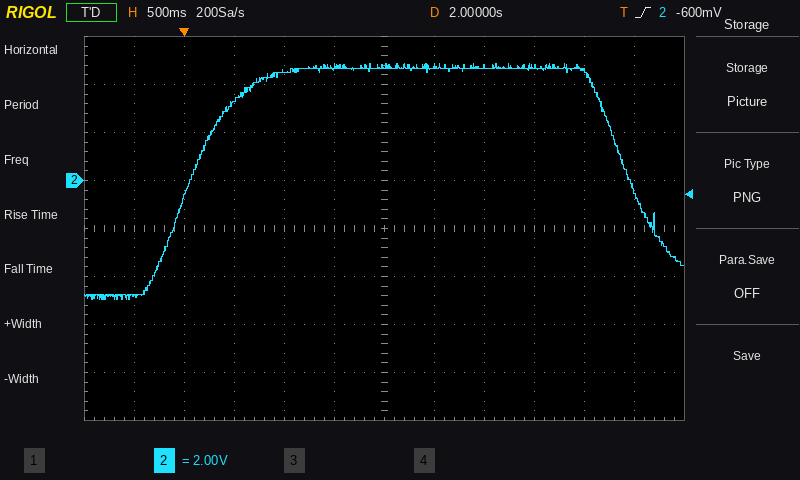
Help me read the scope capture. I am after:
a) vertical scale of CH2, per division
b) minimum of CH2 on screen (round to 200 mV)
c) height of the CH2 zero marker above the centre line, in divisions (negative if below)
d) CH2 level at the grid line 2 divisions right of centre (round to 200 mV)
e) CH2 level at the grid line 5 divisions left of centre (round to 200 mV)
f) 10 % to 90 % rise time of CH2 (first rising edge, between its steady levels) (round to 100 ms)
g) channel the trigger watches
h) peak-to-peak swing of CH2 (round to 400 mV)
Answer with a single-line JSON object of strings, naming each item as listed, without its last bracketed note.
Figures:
{"vertical scale of CH2, per division": "2 V", "minimum of CH2 on screen": "-5.0 V", "height of the CH2 zero marker above the centre line, in divisions": "+1.0 div", "CH2 level at the grid line 2 divisions right of centre": "4.8 V", "CH2 level at the grid line 5 divisions left of centre": "-4.8 V", "10 % to 90 % rise time of CH2 (first rising edge, between its steady levels)": "900 ms", "channel the trigger watches": "CH2", "peak-to-peak swing of CH2": "10.0 V"}
